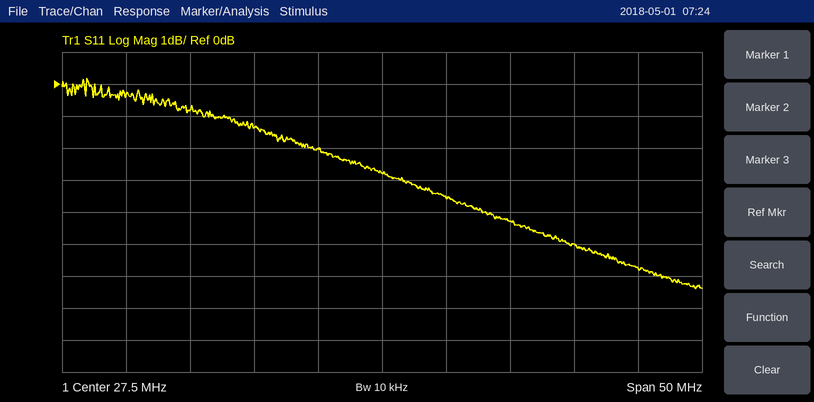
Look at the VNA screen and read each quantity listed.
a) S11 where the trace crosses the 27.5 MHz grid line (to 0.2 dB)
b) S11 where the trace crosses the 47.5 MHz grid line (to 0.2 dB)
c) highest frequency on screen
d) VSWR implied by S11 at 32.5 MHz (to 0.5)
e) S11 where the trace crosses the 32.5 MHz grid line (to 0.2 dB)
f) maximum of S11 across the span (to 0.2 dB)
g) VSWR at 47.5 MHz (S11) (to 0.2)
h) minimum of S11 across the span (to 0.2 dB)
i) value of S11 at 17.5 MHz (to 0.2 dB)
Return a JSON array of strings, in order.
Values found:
["-2.8 dB", "-5.8 dB", "52.5 MHz", "5.0", "-3.6 dB", "0.2 dB", "3.2", "-6.4 dB", "-1.4 dB"]
